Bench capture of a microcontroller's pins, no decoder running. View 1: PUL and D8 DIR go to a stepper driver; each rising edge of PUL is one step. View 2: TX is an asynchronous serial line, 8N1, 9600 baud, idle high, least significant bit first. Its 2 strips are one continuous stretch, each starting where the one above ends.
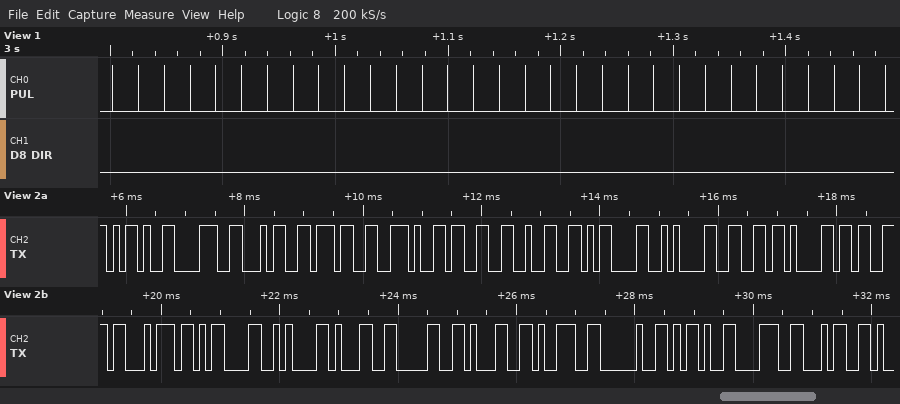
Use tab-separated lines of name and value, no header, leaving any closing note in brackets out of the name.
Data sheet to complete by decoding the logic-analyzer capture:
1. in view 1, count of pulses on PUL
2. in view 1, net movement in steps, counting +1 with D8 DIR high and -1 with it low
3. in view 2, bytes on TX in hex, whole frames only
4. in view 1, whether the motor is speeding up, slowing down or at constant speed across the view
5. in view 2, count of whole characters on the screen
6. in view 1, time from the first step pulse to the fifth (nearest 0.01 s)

in view 1, count of pulses on PUL	31
in view 1, net movement in steps, counting +1 with D8 DIR high and -1 with it low	-31
in view 2, bytes on TX in hex, whole frames only	0x2D 0x38 0x34 0x37 0x2E 0x33 0x32 0x0D 0x0A 0x66 0x61 0x73 0x74 0x0D 0x0A 0x31 0x30 0x31 0x39 0x20 0x2D 0x38 0x34
in view 1, whether the motor is speeding up, slowing down or at constant speed across the view	constant speed
in view 2, count of whole characters on the screen	23
in view 1, time from the first step pulse to the fifth	0.09 s
